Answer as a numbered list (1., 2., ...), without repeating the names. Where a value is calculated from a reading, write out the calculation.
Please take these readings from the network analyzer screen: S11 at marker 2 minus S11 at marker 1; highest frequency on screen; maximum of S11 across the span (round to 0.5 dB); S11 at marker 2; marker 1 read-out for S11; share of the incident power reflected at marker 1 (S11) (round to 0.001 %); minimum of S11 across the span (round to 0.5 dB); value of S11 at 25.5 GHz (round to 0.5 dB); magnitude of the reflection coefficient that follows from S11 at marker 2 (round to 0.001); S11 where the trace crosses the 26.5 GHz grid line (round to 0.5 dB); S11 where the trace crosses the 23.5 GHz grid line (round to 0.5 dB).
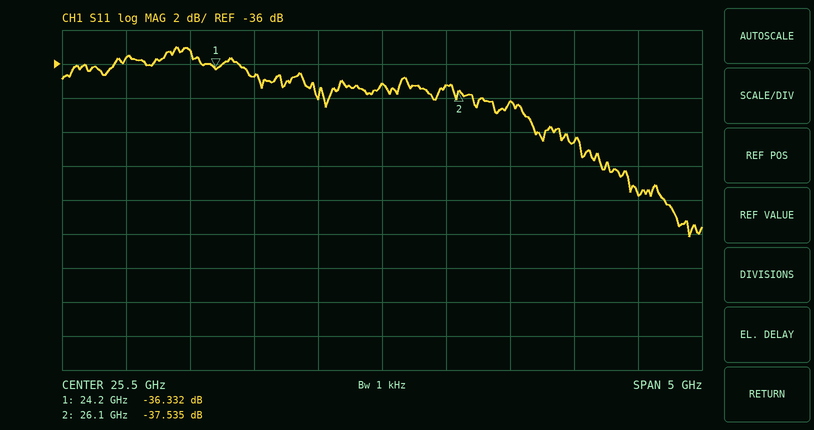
1. -37.535 − (-36.332) = -1.203 dB
2. 28 GHz
3. -35.0 dB
4. -37.535 dB
5. -36.332 dB
6. 10^(-36.332/10) ≈ 0.023 %
7. -46.0 dB
8. -37.0 dB
9. 10^(-37.535/20) ≈ 0.013
10. -38.0 dB
11. -35.5 dB
